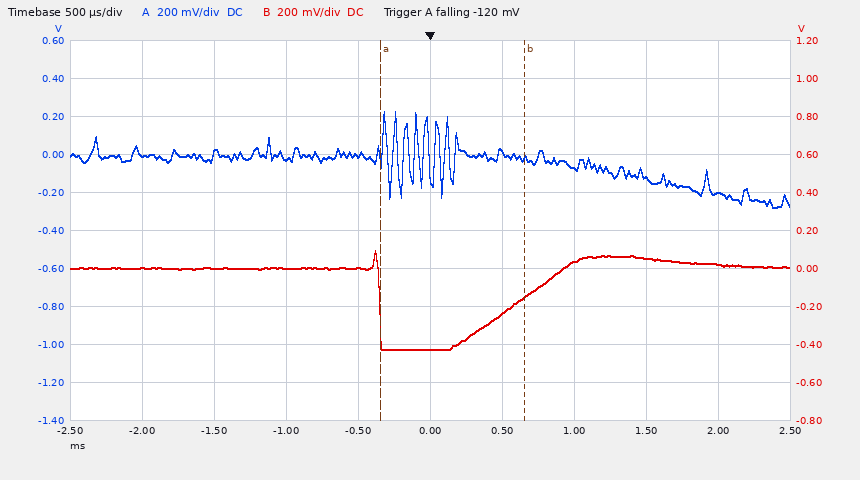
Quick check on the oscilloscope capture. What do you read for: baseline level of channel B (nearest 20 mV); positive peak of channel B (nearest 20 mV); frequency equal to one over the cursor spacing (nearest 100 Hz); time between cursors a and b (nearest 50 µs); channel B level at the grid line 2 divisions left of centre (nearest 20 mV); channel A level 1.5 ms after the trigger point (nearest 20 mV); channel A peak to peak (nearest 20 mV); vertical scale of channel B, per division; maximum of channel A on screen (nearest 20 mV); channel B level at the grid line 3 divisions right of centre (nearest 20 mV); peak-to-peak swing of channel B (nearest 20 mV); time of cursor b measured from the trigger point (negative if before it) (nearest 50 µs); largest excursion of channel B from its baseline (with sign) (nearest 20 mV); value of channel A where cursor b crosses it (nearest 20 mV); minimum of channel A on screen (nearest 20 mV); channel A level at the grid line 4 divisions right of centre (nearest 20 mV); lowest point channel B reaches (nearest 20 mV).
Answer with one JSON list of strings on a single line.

["0 mV", "100 mV", "1.0 kHz", "1.00 ms", "0 mV", "-120 mV", "500 mV", "200 mV", "220 mV", "60 mV", "520 mV", "+650 µs", "-420 mV", "-20 mV", "-280 mV", "-200 mV", "-420 mV"]
